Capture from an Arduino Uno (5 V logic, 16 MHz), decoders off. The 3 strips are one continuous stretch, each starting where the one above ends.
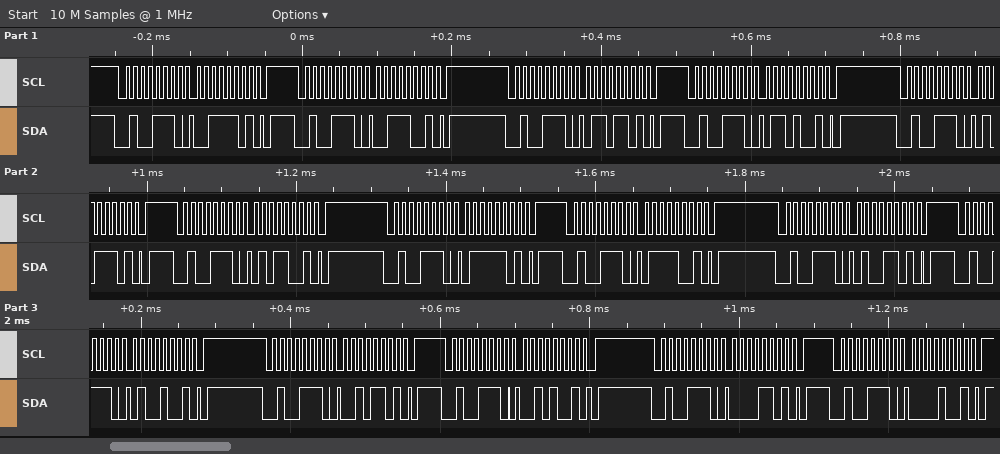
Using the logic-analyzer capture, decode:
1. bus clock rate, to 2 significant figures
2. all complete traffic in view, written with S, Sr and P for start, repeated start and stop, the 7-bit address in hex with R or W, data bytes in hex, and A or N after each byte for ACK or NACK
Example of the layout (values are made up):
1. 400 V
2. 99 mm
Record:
1. 100 kHz
2. S 27W A 3D A P S 27W A 39 A P S 27W A 6D A P S 27W A 69 A P S 27W A 5D A P S 27W A 59 A P S 27W A 7D A P S 27W A 79 A P S 27W A 4D A P S 27W A 49 A P S 27W A 2D A P S 27W A 29 A P S 27W A 0D A P S 27W A 09 A P
